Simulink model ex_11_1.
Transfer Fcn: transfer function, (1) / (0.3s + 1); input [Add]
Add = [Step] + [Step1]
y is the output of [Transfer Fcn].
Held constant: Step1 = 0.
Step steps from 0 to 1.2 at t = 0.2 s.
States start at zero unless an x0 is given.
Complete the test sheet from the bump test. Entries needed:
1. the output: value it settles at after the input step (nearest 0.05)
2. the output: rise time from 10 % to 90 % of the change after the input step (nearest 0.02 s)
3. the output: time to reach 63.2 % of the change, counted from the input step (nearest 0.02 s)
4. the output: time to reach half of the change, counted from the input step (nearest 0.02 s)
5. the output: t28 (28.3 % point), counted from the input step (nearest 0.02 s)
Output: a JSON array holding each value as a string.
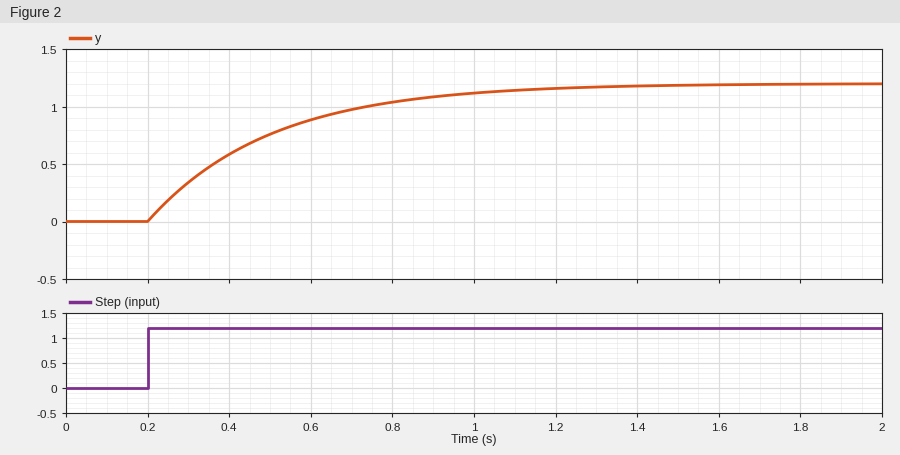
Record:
["1.20", "0.66 s", "0.30 s", "0.20 s", "0.10 s"]
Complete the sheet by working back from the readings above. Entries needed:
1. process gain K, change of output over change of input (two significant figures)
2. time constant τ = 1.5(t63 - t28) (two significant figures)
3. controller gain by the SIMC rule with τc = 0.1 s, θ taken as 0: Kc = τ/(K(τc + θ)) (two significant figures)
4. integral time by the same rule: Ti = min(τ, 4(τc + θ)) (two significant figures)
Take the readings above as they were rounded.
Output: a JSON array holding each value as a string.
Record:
["1.0", "0.30 s", "3.0", "0.30 s"]
